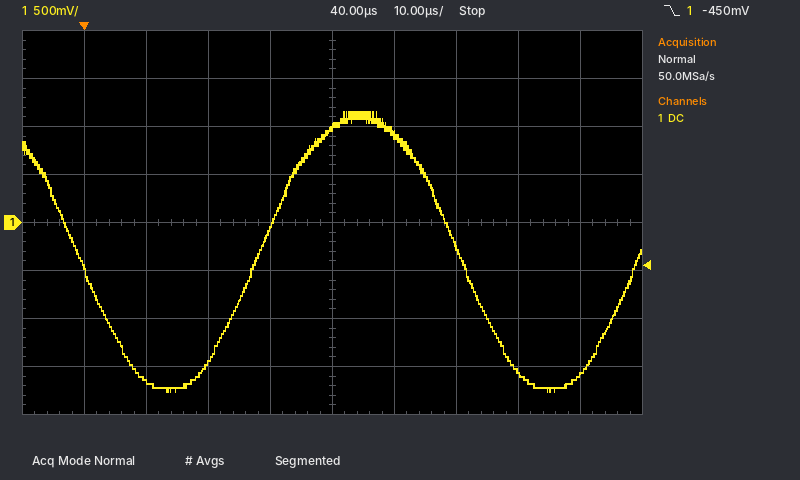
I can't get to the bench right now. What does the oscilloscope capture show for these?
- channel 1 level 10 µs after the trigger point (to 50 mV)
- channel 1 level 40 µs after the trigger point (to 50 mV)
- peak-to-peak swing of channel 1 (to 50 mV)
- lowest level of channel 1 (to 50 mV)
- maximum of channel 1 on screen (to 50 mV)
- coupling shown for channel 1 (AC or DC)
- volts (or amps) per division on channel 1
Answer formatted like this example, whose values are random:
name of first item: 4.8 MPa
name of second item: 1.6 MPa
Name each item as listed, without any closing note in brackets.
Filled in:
channel 1 level 10 µs after the trigger point: -1.65 V
channel 1 level 40 µs after the trigger point: 1.00 V
peak-to-peak swing of channel 1: 2.90 V
lowest level of channel 1: -1.75 V
maximum of channel 1 on screen: 1.15 V
coupling shown for channel 1: DC
volts (or amps) per division on channel 1: 500 mV
